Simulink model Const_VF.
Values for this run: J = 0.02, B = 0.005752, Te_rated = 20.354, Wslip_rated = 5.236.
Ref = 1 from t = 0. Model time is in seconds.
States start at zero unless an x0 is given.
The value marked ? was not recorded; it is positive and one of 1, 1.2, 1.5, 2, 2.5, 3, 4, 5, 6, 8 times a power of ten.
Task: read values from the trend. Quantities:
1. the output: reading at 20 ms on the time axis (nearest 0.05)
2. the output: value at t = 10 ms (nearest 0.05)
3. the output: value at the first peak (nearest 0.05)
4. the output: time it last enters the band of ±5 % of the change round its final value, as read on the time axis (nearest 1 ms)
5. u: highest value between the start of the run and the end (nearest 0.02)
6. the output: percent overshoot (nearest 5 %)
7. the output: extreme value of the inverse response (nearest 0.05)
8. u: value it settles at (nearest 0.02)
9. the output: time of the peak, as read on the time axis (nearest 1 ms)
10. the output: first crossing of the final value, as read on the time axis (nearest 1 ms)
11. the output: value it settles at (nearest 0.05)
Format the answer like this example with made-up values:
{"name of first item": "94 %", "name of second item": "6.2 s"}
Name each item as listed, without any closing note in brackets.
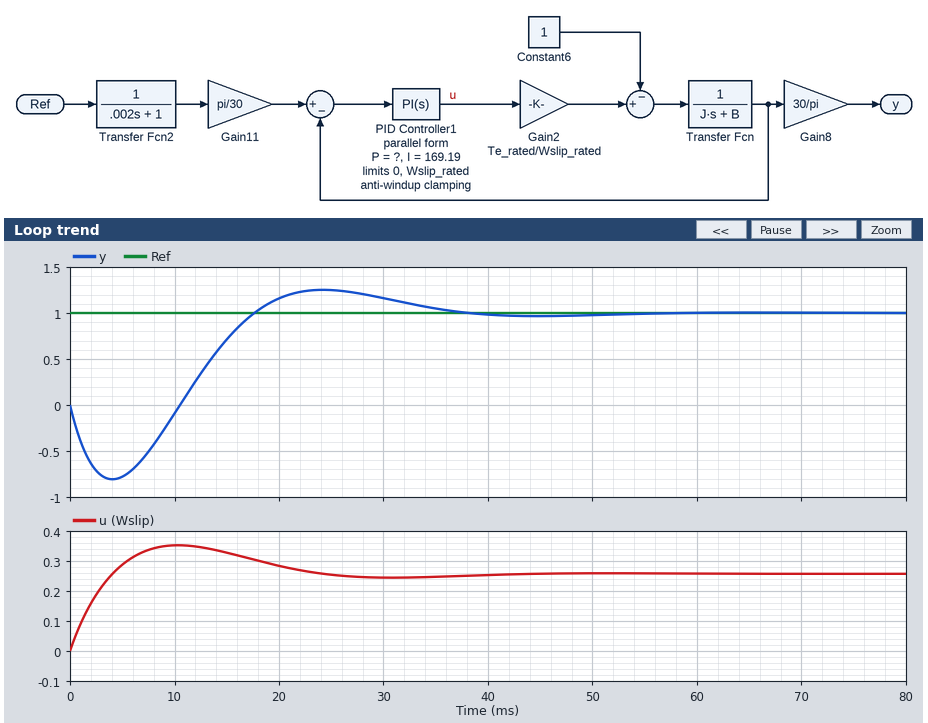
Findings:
{"the output: reading at 20 ms on the time axis": "1.15", "the output: value at t = 10 ms": "-0.10", "the output: value at the first peak": "1.25", "the output: time it last enters the band of ±5 % of the change round its final value, as read on the time axis": "35 ms", "u: highest value between the start of the run and the end": "0.36", "the output: percent overshoot": "25 %", "the output: extreme value of the inverse response": "-0.80", "u: value it settles at": "0.26", "the output: time of the peak, as read on the time axis": "24 ms", "the output: first crossing of the final value, as read on the time axis": "18 ms", "the output: value it settles at": "1.00"}
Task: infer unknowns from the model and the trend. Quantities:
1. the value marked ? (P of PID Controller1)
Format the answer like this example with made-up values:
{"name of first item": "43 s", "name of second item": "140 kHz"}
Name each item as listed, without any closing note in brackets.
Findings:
{"the value marked ?": "1"}
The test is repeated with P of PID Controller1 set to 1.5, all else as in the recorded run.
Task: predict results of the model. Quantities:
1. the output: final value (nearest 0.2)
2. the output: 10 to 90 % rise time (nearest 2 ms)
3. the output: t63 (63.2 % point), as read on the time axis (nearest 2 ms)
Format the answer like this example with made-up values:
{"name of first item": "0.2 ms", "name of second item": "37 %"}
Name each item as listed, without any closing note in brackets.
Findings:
{"the output: final value": "1.0", "the output: 10 to 90 % rise time": "10 ms", "the output: t63 (63.2 % point), as read on the time axis": "14 ms"}
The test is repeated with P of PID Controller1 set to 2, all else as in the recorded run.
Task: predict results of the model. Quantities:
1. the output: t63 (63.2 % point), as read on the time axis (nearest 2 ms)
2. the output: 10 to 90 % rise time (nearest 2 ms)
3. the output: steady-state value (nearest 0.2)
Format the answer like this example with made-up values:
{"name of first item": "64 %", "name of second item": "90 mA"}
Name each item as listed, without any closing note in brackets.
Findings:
{"the output: t63 (63.2 % point), as read on the time axis": "14 ms", "the output: 10 to 90 % rise time": "18 ms", "the output: steady-state value": "1.0"}
